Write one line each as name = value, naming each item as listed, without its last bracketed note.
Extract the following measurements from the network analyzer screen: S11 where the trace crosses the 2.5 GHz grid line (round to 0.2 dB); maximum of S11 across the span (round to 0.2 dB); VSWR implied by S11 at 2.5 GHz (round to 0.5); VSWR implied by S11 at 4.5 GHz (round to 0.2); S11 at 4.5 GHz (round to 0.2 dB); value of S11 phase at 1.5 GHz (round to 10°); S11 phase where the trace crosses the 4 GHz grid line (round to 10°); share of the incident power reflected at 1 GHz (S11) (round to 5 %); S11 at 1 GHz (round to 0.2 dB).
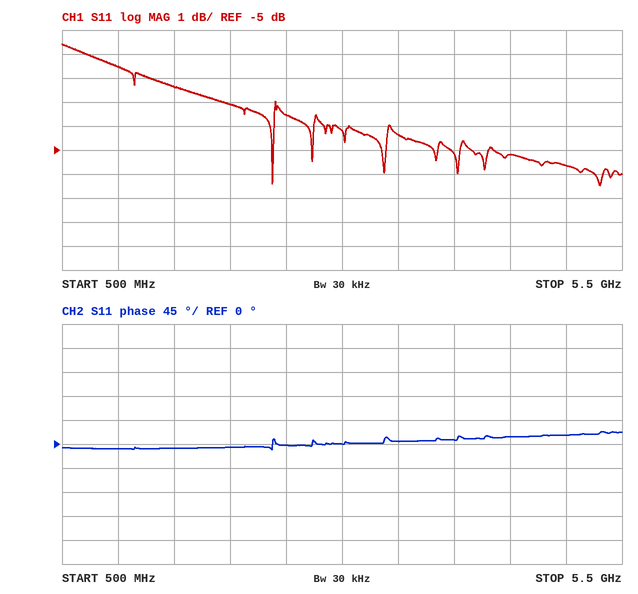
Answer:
S11 where the trace crosses the 2.5 GHz grid line = -3.6 dB
maximum of S11 across the span = -0.6 dB
VSWR implied by S11 at 2.5 GHz = 5.0
VSWR implied by S11 at 4.5 GHz = 3.4
S11 at 4.5 GHz = -5.2 dB
value of S11 phase at 1.5 GHz = -10°
S11 phase where the trace crosses the 4 GHz grid line = 10°
share of the incident power reflected at 1 GHz (S11) = 70 %
S11 at 1 GHz = -1.6 dB
